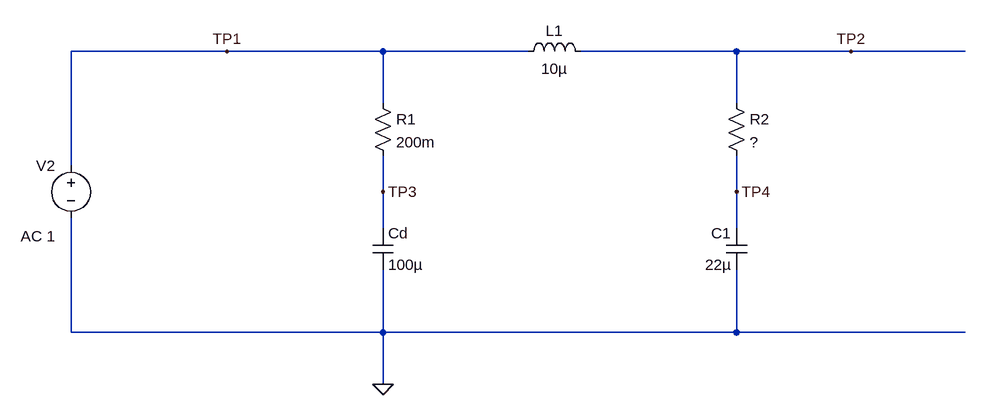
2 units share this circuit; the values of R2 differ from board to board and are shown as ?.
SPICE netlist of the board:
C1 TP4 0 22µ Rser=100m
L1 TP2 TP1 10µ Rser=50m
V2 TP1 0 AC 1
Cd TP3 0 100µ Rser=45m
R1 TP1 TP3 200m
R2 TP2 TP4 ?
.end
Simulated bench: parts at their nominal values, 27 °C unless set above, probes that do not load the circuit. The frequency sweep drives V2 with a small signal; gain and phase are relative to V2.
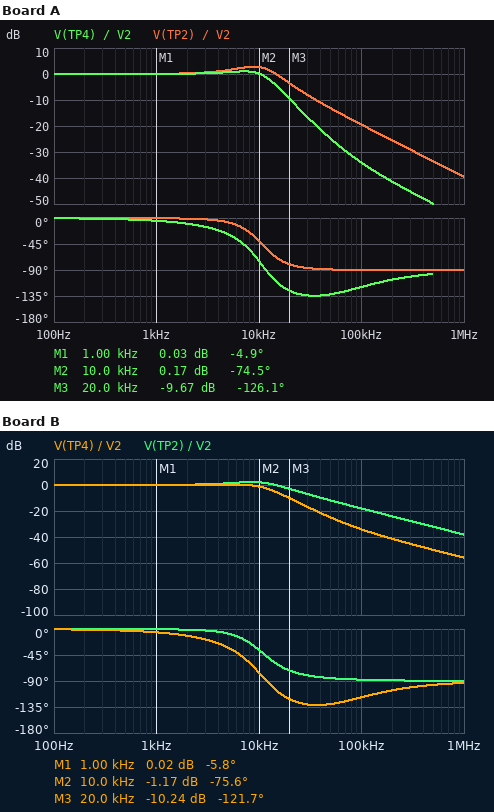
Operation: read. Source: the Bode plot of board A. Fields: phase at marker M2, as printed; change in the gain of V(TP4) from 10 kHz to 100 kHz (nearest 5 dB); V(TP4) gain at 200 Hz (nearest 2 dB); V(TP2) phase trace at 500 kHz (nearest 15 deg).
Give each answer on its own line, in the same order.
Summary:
-74.5 deg
-35 dB
0 dB
-90 deg
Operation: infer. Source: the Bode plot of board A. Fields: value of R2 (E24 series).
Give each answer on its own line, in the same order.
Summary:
0.56 Ω
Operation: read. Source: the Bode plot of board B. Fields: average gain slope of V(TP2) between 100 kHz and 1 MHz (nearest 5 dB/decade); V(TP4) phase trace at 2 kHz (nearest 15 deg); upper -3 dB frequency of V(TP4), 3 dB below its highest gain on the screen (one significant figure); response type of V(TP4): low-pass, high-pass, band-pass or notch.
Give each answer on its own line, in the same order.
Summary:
-20 dB/decade
-15 deg
10 kHz
low-pass
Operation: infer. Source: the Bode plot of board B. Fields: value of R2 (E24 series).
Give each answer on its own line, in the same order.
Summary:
0.68 Ω
